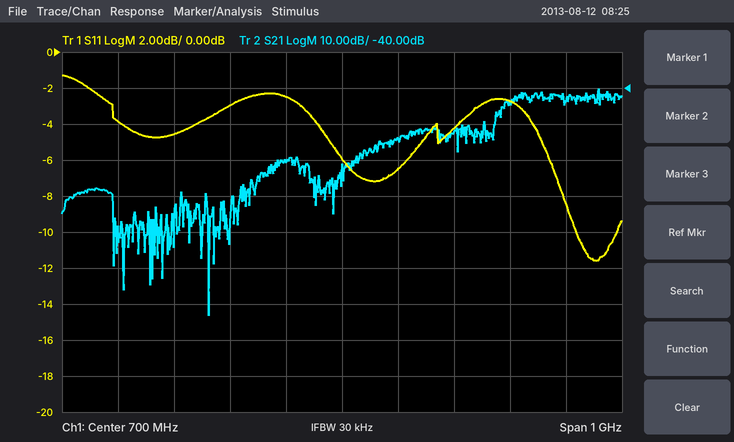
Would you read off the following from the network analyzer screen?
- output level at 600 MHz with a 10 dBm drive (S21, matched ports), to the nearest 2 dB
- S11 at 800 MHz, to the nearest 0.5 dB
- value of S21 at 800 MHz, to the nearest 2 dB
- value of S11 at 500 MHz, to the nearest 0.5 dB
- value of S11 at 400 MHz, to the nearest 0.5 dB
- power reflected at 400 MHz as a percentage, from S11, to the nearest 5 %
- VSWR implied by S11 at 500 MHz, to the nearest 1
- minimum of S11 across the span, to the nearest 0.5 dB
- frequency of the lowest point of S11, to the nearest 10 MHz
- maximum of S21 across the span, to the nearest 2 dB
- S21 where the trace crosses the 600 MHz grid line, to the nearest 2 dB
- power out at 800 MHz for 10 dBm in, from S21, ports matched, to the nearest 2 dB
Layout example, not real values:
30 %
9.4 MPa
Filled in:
-50 dBm
-6.5 dB
-54 dB
-3.0 dB
-4.5 dB
35 %
6
-11.5 dB
1.15 GHz
-40 dB
-60 dB
-44 dBm
